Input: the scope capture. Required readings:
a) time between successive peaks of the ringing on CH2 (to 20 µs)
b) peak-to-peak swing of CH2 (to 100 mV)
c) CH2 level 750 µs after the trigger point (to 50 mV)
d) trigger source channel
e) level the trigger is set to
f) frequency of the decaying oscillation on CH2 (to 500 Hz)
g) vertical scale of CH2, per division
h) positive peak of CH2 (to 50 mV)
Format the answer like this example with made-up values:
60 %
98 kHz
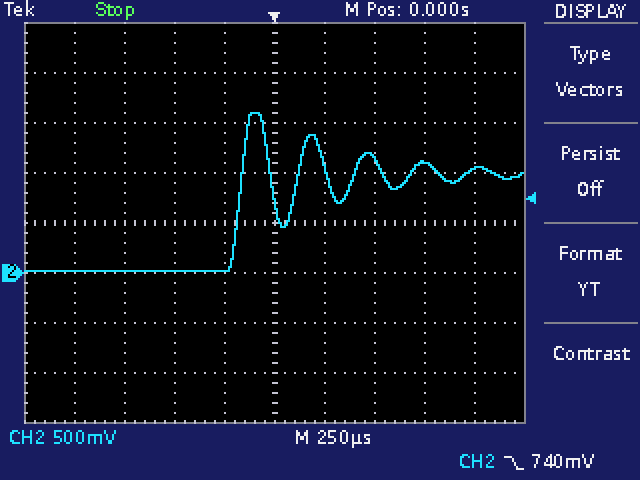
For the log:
280 µs
1.60 V
1.10 V
CH2
740 mV
3.5 kHz
500 mV
1.60 V
